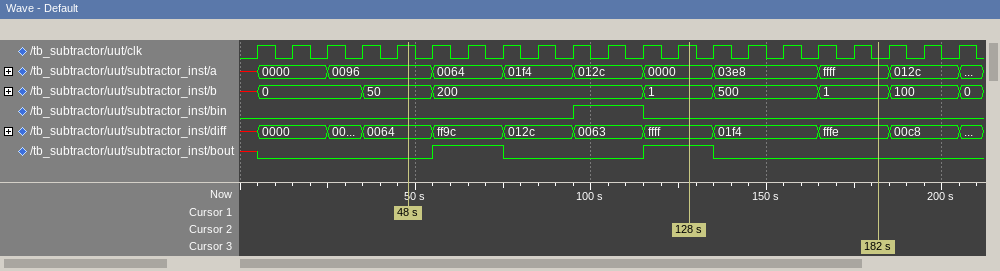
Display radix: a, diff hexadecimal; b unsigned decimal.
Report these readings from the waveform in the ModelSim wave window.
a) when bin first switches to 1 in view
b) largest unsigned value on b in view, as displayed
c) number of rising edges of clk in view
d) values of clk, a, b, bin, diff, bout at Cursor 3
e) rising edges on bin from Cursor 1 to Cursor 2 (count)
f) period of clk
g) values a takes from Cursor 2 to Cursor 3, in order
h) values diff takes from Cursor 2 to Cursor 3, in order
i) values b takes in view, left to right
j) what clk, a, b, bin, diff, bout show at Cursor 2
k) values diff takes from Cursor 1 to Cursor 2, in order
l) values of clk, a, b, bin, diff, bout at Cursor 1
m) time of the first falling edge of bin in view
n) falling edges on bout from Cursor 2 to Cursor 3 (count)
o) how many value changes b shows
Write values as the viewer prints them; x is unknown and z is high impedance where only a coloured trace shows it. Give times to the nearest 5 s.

95 s
500
21
clk=0, a=ffff, b=1, bin=0, diff=fffe, bout=0
1
10 s
0000, 03e8, ffff
ffff, 01f4, fffe
x, 0, 50, 200, 1, 500, 1, 100, 0
clk=1, a=0000, b=1, bin=0, diff=ffff, bout=1
0064, ff9c, 012c, 0063, ffff
clk=1, a=0096, b=50, bin=0, diff=0064, bout=0
115 s
1
8
